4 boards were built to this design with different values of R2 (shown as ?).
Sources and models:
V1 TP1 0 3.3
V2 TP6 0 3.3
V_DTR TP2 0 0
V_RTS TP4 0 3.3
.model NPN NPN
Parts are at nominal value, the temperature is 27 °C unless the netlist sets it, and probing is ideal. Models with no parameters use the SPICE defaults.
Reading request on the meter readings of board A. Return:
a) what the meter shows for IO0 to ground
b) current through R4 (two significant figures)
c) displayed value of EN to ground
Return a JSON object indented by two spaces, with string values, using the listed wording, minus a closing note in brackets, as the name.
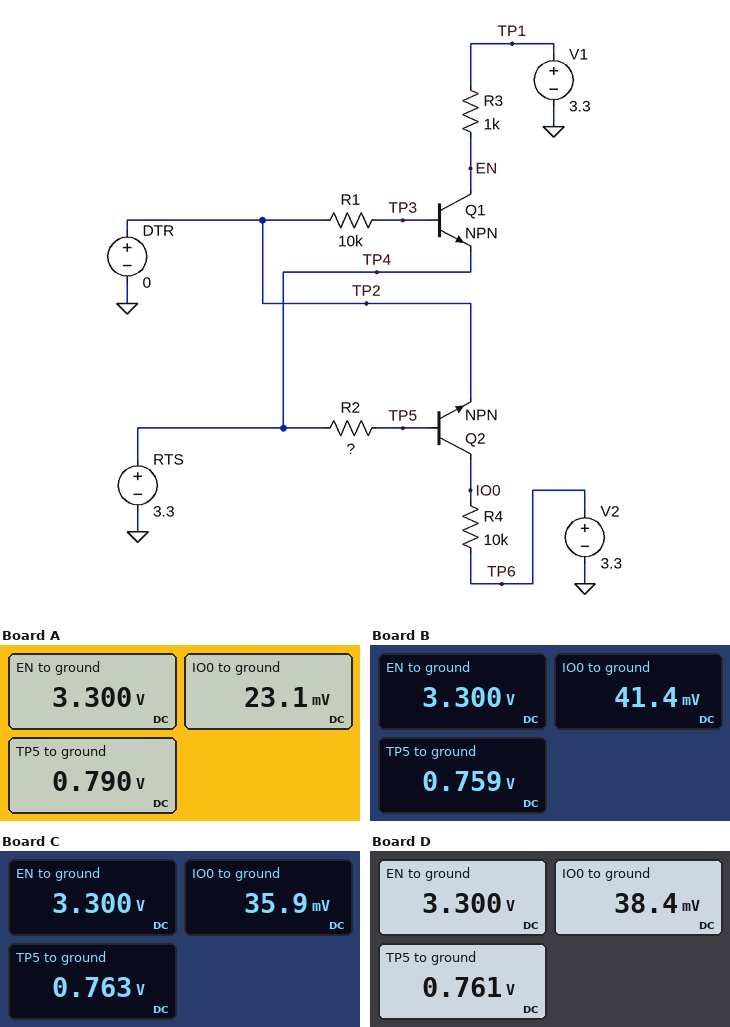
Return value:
{
  "what the meter shows for IO0 to ground": "23.1 mV",
  "current through R4": "330 µA",
  "displayed value of EN to ground": "3.300 V"
}
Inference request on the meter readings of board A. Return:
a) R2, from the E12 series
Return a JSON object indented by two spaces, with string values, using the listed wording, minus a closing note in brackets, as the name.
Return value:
{
  "R2, from the E12 series": "3.3 kΩ"
}
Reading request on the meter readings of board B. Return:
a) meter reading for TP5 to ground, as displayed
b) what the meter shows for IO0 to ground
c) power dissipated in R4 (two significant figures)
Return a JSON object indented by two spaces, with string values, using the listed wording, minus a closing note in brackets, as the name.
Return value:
{
  "meter reading for TP5 to ground, as displayed": "0.759 V",
  "what the meter shows for IO0 to ground": "41.4 mV",
  "power dissipated in R4": "1.1 mW"
}
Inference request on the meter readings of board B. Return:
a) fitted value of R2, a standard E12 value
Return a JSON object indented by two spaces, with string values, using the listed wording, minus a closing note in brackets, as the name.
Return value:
{
  "fitted value of R2, a standard E12 value": "22 kΩ"
}
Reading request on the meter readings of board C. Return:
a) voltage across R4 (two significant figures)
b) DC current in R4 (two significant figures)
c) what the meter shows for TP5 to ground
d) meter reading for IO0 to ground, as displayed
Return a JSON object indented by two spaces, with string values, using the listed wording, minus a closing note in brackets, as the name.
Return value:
{
  "voltage across R4": "3.3 V",
  "DC current in R4": "330 µA",
  "what the meter shows for TP5 to ground": "0.763 V",
  "meter reading for IO0 to ground, as displayed": "35.9 mV"
}
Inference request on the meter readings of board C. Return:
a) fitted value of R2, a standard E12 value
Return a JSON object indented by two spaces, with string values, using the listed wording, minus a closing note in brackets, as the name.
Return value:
{
  "fitted value of R2, a standard E12 value": "15 kΩ"
}
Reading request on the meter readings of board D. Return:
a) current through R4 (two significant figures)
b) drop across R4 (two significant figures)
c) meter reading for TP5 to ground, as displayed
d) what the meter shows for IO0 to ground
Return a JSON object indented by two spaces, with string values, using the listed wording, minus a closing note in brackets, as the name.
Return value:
{
  "current through R4": "330 µA",
  "drop across R4": "3.3 V",
  "meter reading for TP5 to ground, as displayed": "0.761 V",
  "what the meter shows for IO0 to ground": "38.4 mV"
}
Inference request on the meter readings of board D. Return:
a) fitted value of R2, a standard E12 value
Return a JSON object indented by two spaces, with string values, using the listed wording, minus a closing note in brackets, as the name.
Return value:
{
  "fitted value of R2, a standard E12 value": "18 kΩ"
}
